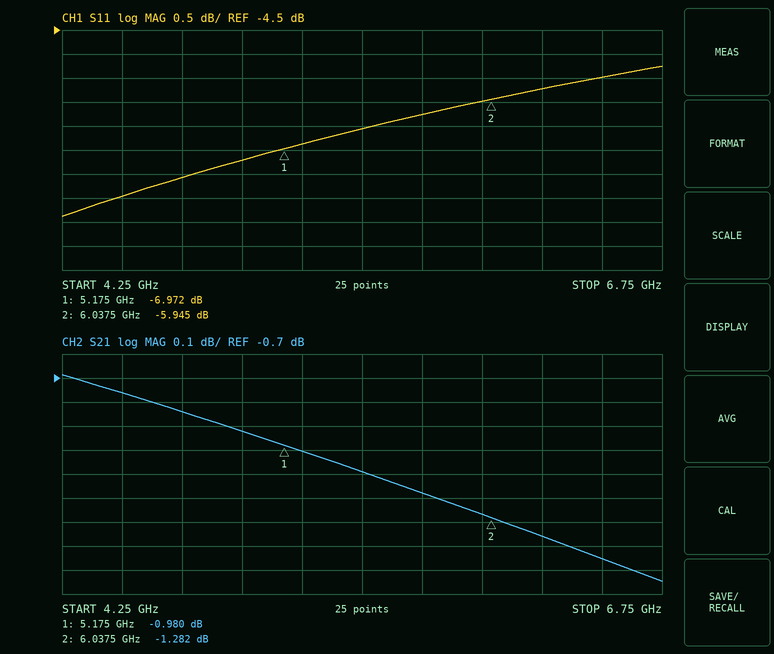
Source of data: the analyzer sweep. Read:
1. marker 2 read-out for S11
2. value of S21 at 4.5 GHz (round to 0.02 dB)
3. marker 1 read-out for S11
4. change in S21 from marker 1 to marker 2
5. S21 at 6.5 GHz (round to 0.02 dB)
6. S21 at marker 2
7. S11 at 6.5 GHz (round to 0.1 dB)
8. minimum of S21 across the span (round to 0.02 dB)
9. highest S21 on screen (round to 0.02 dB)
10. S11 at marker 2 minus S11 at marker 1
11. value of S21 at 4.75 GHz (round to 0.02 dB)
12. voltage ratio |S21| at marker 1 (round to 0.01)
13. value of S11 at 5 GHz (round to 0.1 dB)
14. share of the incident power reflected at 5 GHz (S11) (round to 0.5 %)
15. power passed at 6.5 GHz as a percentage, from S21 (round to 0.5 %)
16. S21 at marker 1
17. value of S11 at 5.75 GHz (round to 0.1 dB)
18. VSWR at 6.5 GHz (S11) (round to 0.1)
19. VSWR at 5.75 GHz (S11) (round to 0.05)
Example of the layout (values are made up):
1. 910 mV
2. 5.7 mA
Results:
1. -5.945 dB
2. -0.76 dB
3. -6.972 dB
4. -0.302 dB
5. -1.46 dB
6. -1.282 dB
7. -5.5 dB
8. -1.54 dB
9. -0.68 dB
10. 1.027 dB
11. -0.84 dB
12. 0.89
13. -7.2 dB
14. 19.0 %
15. 71.5 %
16. -0.980 dB
17. -6.3 dB
18. 3.3
19. 2.90
